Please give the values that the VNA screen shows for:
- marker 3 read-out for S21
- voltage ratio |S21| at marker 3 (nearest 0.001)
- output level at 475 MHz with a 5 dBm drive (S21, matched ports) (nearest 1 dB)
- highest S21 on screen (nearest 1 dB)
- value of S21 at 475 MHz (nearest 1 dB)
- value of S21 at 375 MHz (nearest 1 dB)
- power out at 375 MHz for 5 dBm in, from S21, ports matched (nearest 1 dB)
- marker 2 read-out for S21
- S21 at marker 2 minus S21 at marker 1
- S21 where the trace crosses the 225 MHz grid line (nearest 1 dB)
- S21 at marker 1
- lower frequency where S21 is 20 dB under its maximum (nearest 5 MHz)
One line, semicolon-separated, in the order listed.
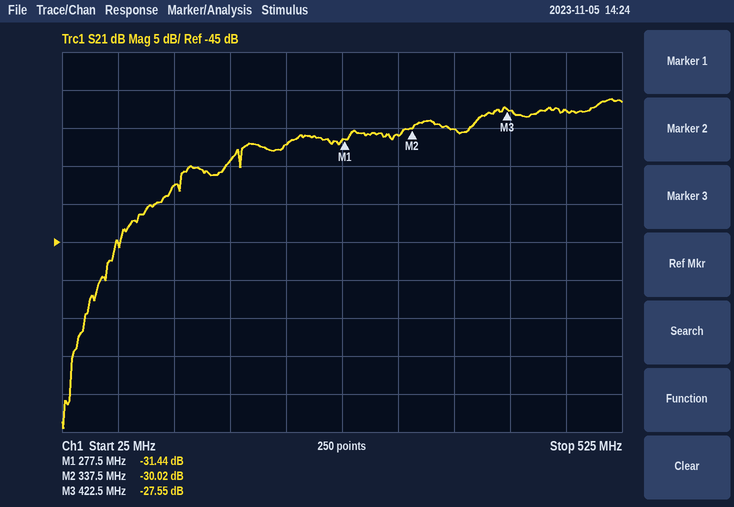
-27.55 dB; 0.042; -23 dBm; -26 dB; -28 dB; -30 dB; -25 dBm; -30.02 dB; 1.42 dB; -32 dB; -31.44 dB; 70 MHz
